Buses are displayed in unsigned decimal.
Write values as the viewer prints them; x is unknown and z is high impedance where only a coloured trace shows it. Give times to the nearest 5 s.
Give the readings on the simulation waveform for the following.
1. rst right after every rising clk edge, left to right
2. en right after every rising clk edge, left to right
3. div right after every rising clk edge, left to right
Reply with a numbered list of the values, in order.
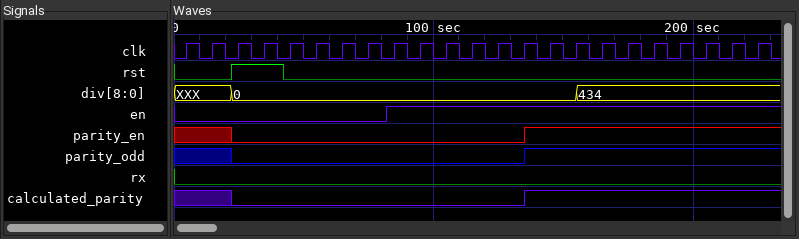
1. 0 0 1 1 0 0 0 0 0 0 0 0 0 0 0 0 0 0 0 0 0 0 0
2. 0 0 0 0 0 0 0 0 1 1 1 1 1 1 1 1 1 1 1 1 1 1 1
3. XXX, XXX, 0, 0, 0, 0, 0, 0, 0, 0, 0, 0, 0, 0, 0, 434, 434, 434, 434, 434, 434, 434, 434
